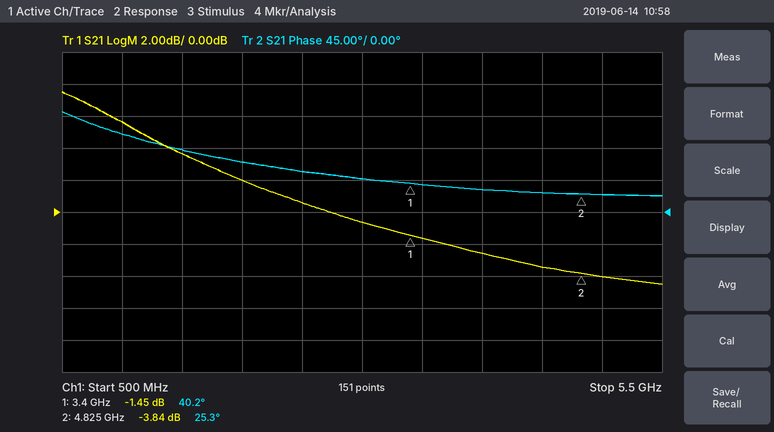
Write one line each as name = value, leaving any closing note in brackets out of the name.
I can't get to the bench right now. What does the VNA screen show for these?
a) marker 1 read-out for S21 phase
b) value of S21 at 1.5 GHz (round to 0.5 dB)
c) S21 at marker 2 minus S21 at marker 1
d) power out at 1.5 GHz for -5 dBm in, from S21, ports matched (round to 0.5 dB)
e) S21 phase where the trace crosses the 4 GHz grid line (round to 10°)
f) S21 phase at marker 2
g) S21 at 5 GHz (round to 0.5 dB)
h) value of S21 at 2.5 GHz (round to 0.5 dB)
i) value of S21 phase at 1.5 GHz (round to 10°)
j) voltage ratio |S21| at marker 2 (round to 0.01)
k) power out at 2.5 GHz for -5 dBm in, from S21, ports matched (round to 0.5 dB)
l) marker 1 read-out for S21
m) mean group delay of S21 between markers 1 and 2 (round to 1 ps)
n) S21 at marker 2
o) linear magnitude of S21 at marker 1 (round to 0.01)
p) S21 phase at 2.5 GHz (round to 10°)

marker 1 read-out for S21 phase = 40.2°
value of S21 at 1.5 GHz = 3.5 dB
S21 at marker 2 minus S21 at marker 1 = -2.39 dB
power out at 1.5 GHz for -5 dBm in, from S21, ports matched = -1.5 dBm
S21 phase where the trace crosses the 4 GHz grid line = 30°
S21 phase at marker 2 = 25.3°
S21 at 5 GHz = -4.0 dB
value of S21 at 2.5 GHz = 0.5 dB
value of S21 phase at 1.5 GHz = 90°
voltage ratio |S21| at marker 2 = 0.64
power out at 2.5 GHz for -5 dBm in, from S21, ports matched = -4.5 dBm
marker 1 read-out for S21 = -1.45 dB
mean group delay of S21 between markers 1 and 2 = 29 ps
S21 at marker 2 = -3.84 dB
linear magnitude of S21 at marker 1 = 0.85
S21 phase at 2.5 GHz = 60°
